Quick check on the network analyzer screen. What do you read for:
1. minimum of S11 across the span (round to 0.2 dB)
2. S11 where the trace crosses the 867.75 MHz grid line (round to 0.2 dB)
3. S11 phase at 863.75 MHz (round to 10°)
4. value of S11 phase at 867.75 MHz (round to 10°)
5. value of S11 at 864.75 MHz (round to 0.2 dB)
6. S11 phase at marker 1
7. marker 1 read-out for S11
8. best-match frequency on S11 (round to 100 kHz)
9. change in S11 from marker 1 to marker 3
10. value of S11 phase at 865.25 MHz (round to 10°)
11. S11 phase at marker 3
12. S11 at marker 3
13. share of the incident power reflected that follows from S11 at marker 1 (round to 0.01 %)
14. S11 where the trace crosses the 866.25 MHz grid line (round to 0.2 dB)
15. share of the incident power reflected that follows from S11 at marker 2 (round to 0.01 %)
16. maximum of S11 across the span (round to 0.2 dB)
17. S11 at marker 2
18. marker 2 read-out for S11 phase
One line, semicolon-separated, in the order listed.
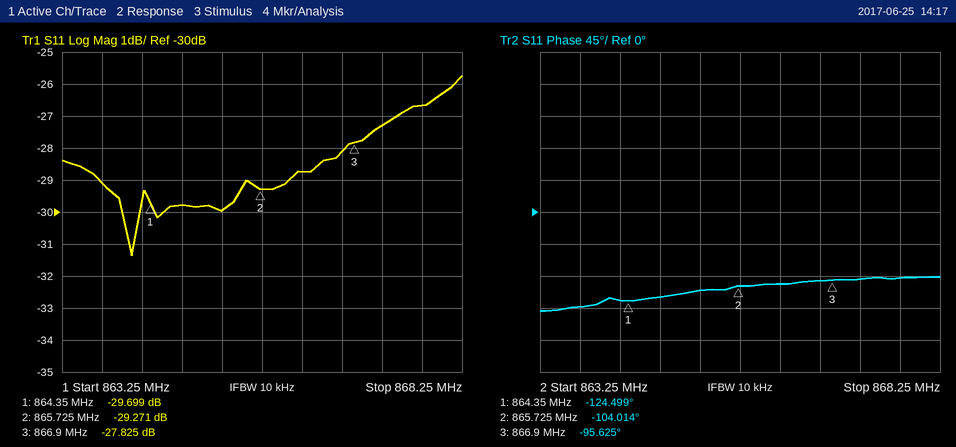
-31.4 dB; -26.6 dB; -130°; -90°; -29.8 dB; -124.499°; -29.699 dB; 864.1 MHz; 1.874 dB; -110°; -95.625°; -27.825 dB; 0.11 %; -28.8 dB; 0.12 %; -25.8 dB; -29.271 dB; -104.014°
